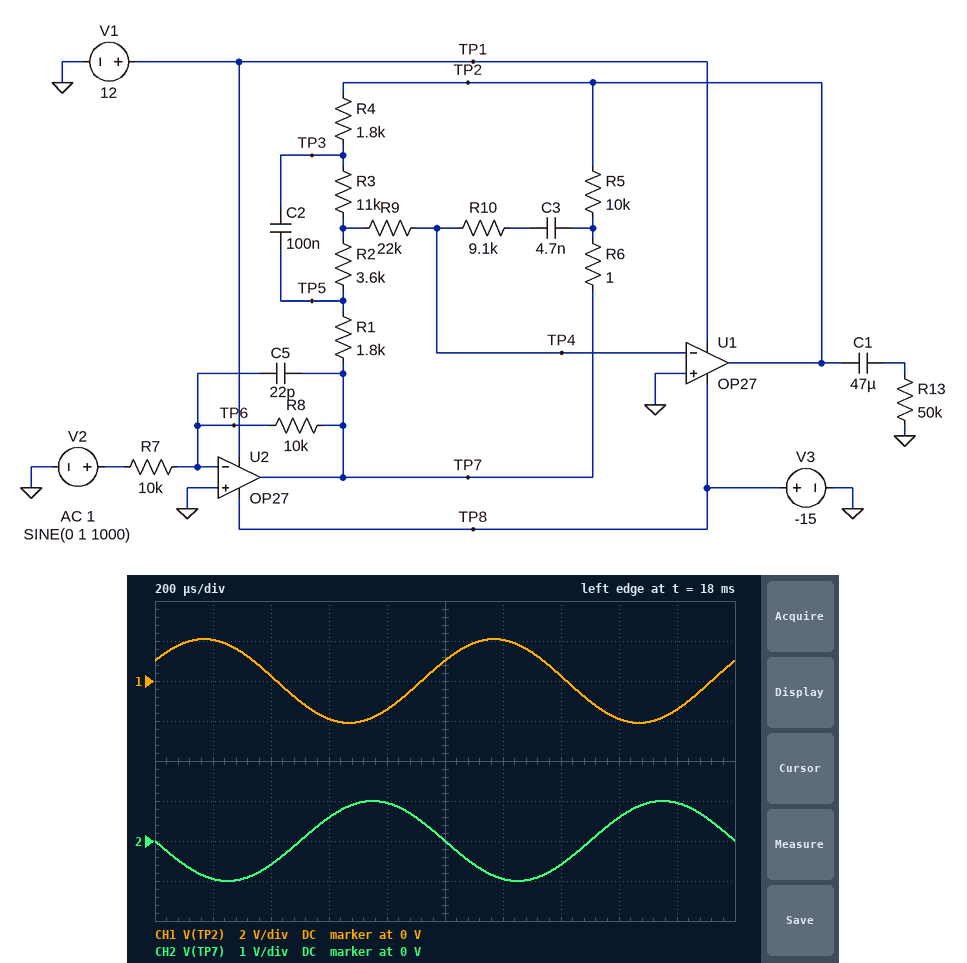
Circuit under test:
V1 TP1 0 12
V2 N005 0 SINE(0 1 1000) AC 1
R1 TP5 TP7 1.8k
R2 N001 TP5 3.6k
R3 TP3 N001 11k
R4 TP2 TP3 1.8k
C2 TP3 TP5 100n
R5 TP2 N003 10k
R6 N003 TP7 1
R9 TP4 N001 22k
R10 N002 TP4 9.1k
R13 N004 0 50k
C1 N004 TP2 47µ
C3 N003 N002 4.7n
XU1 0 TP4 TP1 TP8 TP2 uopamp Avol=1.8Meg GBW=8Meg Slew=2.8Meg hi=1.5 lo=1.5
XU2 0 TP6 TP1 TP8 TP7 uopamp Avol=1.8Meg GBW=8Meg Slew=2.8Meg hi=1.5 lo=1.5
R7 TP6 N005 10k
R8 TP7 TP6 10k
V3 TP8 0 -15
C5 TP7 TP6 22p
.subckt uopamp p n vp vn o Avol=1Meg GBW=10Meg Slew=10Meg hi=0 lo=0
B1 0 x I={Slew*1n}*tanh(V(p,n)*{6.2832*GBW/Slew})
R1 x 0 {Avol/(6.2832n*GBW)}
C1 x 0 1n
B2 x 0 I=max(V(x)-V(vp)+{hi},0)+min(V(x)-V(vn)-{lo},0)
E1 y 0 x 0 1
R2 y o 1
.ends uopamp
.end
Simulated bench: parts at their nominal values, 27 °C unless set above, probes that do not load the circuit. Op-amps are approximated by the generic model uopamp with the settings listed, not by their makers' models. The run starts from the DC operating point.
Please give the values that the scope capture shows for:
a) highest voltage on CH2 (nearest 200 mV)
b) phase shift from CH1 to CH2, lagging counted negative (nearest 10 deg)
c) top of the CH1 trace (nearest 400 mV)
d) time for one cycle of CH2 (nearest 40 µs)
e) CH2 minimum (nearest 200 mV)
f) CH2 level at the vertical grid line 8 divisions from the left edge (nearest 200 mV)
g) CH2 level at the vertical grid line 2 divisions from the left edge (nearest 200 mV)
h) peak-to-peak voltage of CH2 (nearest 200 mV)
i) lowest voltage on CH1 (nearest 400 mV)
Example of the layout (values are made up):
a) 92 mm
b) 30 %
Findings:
a) 1.0 V
b) 150 deg
c) 2.0 V
d) 1.00 ms
e) -1.0 V
f) 600 mV
g) -600 mV
h) 2.0 V
i) -2.0 V
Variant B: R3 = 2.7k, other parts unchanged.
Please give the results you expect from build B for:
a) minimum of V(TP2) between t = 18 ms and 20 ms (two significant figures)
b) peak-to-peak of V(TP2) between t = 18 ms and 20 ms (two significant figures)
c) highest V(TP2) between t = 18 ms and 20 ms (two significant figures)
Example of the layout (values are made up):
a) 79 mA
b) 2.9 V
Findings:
a) -1.9 V
b) 3.7 V
c) 1.9 V
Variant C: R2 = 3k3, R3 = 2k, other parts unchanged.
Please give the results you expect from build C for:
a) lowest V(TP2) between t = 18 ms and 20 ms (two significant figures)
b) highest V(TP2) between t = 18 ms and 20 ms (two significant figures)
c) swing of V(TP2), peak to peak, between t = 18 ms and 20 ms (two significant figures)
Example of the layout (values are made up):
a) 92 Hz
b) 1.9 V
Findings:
a) -1.8 V
b) 1.8 V
c) 3.6 V
